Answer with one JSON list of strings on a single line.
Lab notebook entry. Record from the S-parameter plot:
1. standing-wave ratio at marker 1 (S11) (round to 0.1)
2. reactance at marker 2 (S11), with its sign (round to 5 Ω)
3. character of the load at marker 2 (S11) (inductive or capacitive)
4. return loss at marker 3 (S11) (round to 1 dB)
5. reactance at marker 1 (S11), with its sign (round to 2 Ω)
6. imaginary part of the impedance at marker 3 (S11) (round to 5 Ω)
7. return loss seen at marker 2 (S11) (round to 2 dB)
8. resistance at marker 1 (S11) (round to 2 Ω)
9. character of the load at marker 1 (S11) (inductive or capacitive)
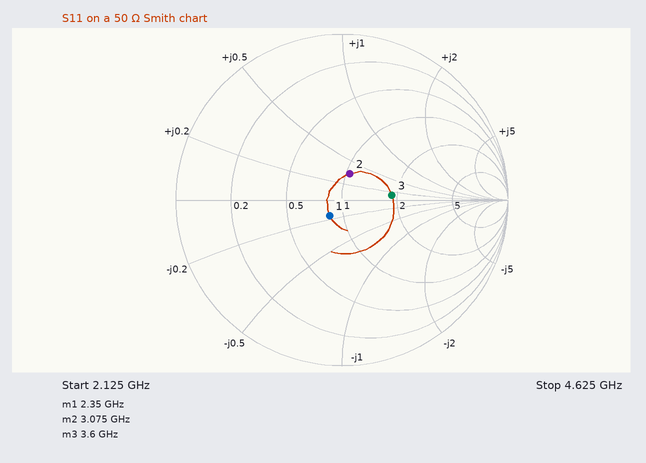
["1.3", "+15 Ω", "inductive", "10 dB", "-8 Ω", "+5 Ω", "16 dB", "42 Ω", "capacitive"]
